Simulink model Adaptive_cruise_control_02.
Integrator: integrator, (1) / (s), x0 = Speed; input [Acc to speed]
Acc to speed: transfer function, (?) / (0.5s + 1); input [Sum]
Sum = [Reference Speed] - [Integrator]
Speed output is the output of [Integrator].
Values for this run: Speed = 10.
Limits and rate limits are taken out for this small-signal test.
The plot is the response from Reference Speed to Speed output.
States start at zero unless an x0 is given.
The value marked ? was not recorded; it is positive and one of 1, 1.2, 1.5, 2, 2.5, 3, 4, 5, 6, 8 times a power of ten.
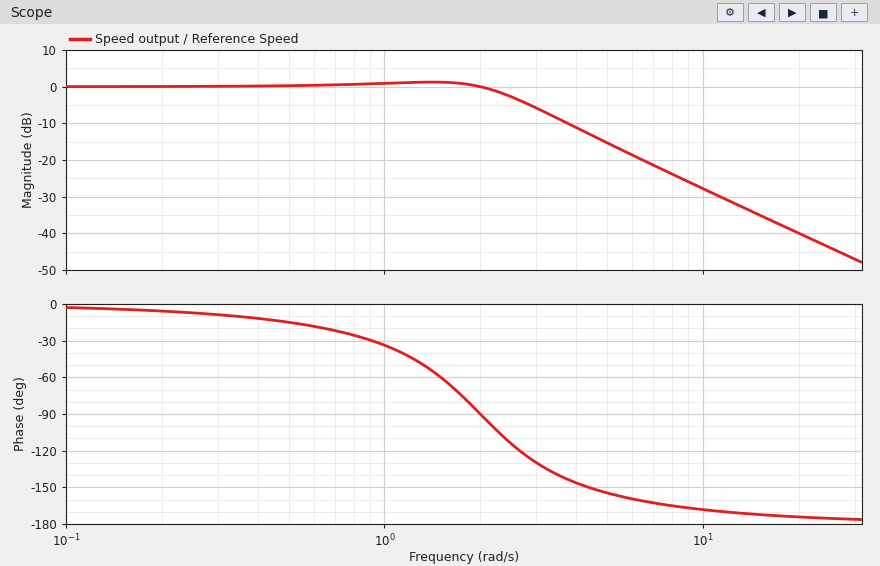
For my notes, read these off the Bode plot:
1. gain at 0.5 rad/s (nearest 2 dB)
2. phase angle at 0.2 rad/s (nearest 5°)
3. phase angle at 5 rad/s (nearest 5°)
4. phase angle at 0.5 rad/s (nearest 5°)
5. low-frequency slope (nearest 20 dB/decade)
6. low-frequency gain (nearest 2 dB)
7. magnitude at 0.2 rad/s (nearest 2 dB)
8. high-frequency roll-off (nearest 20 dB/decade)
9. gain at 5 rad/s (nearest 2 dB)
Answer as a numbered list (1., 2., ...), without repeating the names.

1. 0 dB
2. -5°
3. -155°
4. -15°
5. 0 dB/decade
6. 0 dB
7. 0 dB
8. -40 dB/decade
9. -16 dB
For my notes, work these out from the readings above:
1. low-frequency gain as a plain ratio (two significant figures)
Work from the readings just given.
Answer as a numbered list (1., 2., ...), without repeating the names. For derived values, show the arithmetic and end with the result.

1. 10^(0 / 20) = 1.0
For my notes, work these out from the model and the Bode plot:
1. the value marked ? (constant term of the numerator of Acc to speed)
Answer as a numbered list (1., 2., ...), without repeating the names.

1. 2
